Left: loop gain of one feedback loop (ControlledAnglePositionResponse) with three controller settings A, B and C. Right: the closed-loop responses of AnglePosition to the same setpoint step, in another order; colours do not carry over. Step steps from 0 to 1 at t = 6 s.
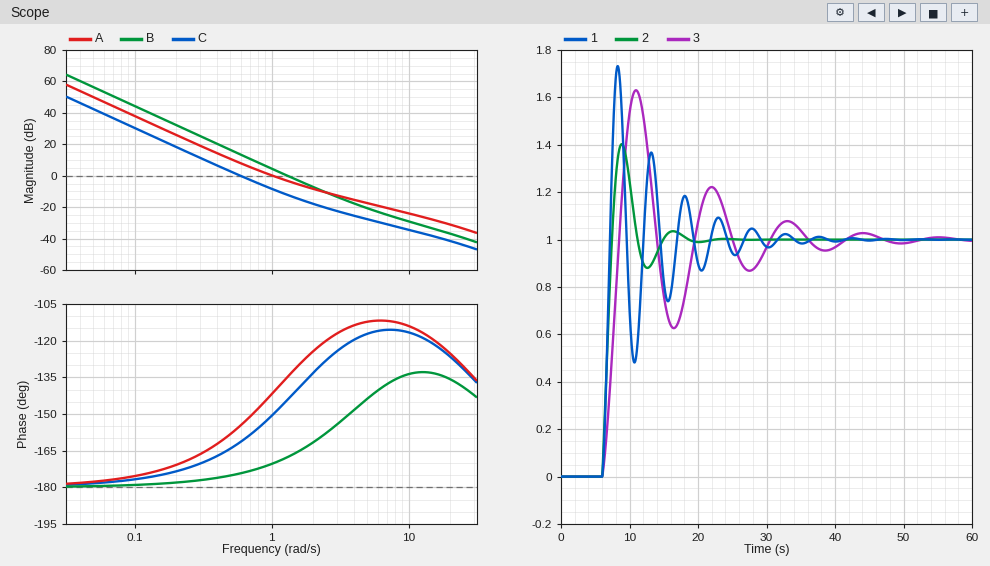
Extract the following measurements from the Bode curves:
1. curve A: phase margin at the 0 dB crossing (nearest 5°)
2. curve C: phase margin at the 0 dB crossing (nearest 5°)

40°
20°
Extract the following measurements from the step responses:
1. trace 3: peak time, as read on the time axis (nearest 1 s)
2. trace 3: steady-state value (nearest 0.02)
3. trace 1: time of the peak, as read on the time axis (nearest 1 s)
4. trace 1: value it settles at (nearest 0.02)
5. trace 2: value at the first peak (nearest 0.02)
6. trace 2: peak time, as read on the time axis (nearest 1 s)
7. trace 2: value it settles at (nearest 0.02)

11 s
1.00
8 s
1.00
1.40
9 s
1.00
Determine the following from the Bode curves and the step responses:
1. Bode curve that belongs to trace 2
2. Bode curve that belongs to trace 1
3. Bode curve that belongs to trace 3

A
B
C
